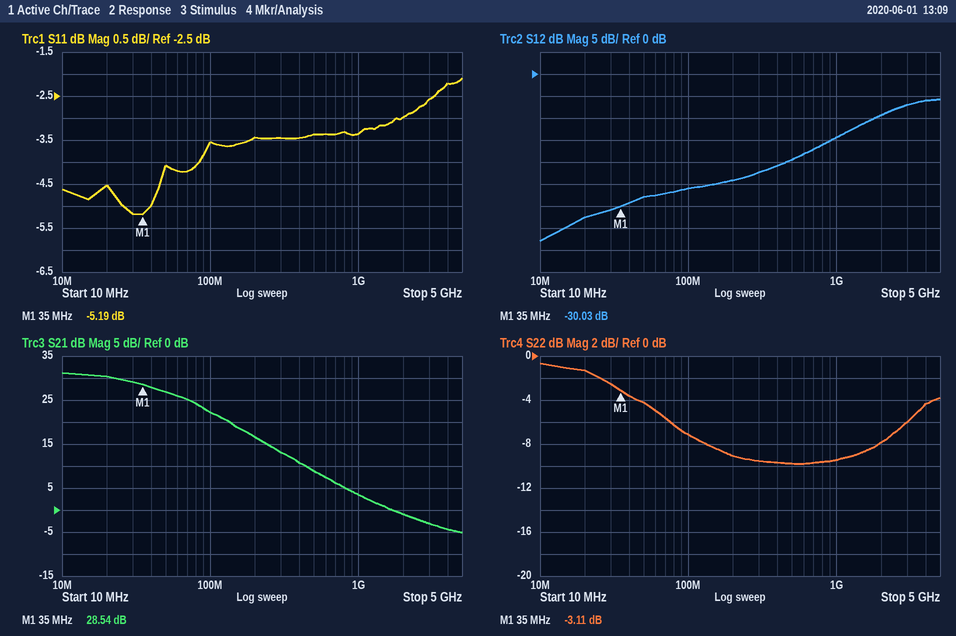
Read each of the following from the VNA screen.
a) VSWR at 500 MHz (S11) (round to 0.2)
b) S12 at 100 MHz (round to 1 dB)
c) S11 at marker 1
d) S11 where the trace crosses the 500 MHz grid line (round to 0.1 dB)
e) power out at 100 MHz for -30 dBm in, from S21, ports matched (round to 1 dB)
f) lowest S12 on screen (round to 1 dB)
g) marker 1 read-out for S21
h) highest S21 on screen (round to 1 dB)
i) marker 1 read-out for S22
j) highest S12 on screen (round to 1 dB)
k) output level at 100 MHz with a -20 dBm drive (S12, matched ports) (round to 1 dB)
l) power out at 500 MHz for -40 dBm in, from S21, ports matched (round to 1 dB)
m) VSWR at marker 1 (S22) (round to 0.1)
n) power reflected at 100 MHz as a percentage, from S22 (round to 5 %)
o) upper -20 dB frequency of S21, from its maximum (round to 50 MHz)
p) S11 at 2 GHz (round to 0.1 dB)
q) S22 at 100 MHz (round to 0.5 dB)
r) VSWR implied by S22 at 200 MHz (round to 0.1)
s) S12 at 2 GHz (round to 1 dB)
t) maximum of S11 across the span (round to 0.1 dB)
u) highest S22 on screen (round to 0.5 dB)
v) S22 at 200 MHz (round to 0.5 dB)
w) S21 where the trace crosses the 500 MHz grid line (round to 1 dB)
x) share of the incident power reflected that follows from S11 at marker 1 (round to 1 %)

5.2
-26 dB
-5.19 dB
-3.4 dB
-8 dBm
-38 dB
28.54 dB
31 dB
-3.11 dB
-6 dB
-46 dBm
-31 dBm
5.6
20 %
400 MHz
-3.0 dB
-7.0 dB
2.1
-9 dB
-2.1 dB
-0.5 dB
-9.0 dB
9 dB
30 %
